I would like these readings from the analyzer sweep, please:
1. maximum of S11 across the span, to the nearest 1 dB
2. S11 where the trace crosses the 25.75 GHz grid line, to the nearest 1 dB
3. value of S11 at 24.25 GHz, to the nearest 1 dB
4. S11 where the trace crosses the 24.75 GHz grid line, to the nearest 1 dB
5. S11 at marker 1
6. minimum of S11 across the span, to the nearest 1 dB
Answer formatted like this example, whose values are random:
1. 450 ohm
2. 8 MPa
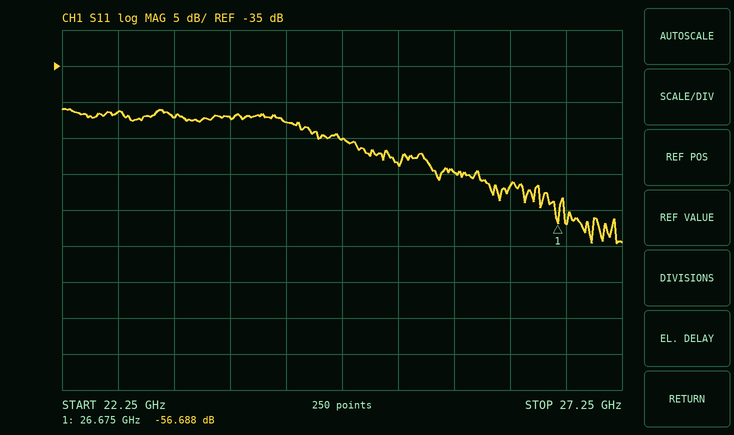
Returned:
1. -41 dB
2. -50 dB
3. -43 dB
4. -45 dB
5. -56.688 dB
6. -60 dB
